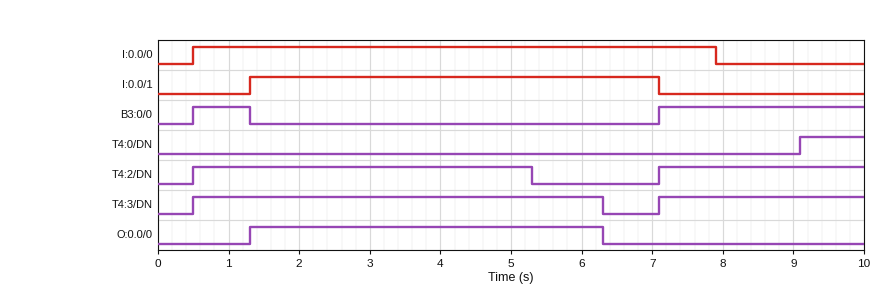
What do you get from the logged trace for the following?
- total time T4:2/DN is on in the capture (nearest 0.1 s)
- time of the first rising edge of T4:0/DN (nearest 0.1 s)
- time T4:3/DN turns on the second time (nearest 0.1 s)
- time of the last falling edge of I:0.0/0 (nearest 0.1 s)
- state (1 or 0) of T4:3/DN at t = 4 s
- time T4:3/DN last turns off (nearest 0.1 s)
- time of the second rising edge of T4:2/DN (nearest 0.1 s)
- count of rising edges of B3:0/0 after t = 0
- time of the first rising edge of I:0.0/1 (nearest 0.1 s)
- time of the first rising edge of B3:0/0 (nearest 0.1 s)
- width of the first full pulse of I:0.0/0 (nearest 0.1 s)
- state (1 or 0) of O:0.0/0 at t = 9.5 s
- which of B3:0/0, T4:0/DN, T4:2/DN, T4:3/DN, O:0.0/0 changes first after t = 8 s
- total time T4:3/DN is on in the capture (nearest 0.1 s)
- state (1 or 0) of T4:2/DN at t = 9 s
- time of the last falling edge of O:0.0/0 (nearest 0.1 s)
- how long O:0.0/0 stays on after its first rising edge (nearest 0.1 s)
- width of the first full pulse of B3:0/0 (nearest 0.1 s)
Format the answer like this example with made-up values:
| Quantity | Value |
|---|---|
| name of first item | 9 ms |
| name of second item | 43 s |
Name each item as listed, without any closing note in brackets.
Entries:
| Quantity | Value |
|---|---|
| total time T4:2/DN is on in the capture | 7.7 s |
| time of the first rising edge of T4:0/DN | 9.1 s |
| time T4:3/DN turns on the second time | 7.1 s |
| time of the last falling edge of I:0.0/0 | 7.9 s |
| state (1 or 0) of T4:3/DN at t = 4 s | 1 |
| time T4:3/DN last turns off | 6.3 s |
| time of the second rising edge of T4:2/DN | 7.1 s |
| count of rising edges of B3:0/0 after t = 0 | 2 |
| time of the first rising edge of I:0.0/1 | 1.3 s |
| time of the first rising edge of B3:0/0 | 0.5 s |
| width of the first full pulse of I:0.0/0 | 7.4 s |
| state (1 or 0) of O:0.0/0 at t = 9.5 s | 0 |
| which of B3:0/0, T4:0/DN, T4:2/DN, T4:3/DN, O:0.0/0 changes first after t = 8 s | T4:0/DN |
| total time T4:3/DN is on in the capture | 8.7 s |
| state (1 or 0) of T4:2/DN at t = 9 s | 1 |
| time of the last falling edge of O:0.0/0 | 6.3 s |
| how long O:0.0/0 stays on after its first rising edge | 5.0 s |
| width of the first full pulse of B3:0/0 | 0.8 s |
